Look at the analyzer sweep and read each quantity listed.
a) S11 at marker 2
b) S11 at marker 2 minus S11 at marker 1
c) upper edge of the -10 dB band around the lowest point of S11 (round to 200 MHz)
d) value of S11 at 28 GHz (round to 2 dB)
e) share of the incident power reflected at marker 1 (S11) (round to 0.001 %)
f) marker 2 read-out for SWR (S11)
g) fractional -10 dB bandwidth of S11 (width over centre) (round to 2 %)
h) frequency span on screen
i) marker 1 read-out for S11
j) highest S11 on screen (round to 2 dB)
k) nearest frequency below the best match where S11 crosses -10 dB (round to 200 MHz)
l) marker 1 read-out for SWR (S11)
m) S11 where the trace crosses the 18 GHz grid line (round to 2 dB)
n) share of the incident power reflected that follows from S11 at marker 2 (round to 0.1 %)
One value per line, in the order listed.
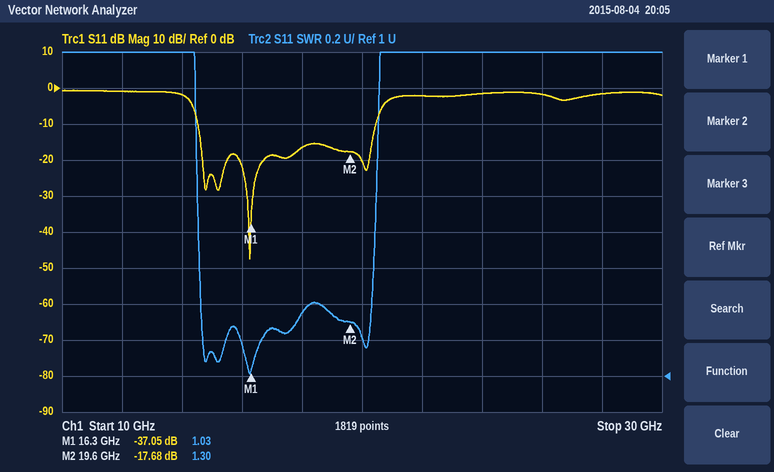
-17.68 dB
19.37 dB
20.4 GHz
-2 dB
0.020 %
1.30
34 %
20 GHz
-37.05 dB
0 dB
14.6 GHz
1.03
-16 dB
1.7 %
